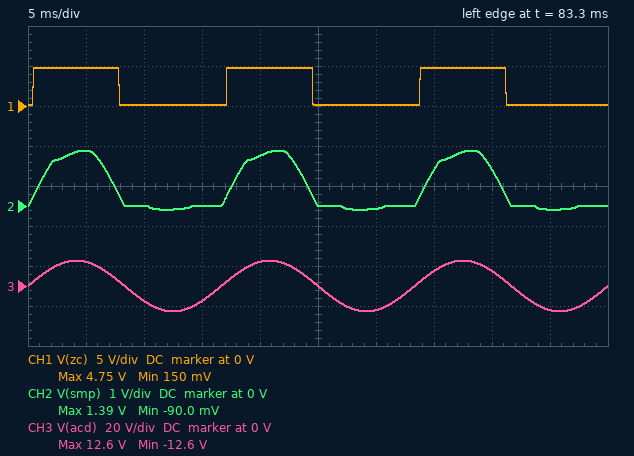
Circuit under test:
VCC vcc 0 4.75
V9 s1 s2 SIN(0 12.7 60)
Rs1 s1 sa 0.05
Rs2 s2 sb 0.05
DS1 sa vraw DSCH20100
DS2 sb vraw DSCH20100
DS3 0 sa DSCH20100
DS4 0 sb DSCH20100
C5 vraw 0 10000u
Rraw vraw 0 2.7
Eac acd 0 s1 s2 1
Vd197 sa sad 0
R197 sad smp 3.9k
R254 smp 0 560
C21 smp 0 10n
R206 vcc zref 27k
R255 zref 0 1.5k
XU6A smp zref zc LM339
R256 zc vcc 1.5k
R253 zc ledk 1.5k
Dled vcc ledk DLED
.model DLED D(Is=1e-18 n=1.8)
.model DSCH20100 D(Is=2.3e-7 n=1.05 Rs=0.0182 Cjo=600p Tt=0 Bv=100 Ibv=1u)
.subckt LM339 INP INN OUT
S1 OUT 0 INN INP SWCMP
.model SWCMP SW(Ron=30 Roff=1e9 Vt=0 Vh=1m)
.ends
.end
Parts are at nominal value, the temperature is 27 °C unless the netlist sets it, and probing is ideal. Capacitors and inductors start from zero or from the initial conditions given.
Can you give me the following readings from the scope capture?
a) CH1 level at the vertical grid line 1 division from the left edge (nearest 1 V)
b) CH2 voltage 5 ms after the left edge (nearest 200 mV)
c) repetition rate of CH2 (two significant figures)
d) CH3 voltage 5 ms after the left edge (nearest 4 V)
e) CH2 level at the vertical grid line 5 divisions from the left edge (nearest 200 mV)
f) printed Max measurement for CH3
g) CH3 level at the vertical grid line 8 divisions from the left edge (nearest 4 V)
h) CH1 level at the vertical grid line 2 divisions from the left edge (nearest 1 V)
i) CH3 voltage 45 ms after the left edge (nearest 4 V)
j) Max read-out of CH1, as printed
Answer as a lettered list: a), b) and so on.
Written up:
a) 5 V
b) 1.4 V
c) 60 Hz
d) 12 V
e) 0 V
f) 12.6 V
g) 8 V
h) 0 V
i) -12 V
j) 4.75 V
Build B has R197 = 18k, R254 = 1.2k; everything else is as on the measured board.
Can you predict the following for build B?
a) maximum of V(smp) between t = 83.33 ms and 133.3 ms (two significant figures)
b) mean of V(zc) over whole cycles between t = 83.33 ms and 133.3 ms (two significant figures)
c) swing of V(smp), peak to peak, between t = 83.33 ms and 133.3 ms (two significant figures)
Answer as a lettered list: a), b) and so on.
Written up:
a) 690 mV
b) 2.0 V
c) 740 mV
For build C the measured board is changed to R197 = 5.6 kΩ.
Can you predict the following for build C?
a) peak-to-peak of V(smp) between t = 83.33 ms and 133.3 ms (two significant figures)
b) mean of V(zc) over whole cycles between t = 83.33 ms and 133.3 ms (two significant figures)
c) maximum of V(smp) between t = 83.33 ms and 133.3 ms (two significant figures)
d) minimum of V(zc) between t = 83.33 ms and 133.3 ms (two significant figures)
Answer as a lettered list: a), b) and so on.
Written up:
a) 1.1 V
b) 2.1 V
c) 1.0 V
d) 150 mV
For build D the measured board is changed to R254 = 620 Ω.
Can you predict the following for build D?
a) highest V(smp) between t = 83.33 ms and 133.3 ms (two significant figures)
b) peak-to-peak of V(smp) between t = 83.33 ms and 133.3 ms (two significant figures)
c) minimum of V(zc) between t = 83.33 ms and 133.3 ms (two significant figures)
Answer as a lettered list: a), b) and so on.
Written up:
a) 1.5 V
b) 1.6 V
c) 150 mV
